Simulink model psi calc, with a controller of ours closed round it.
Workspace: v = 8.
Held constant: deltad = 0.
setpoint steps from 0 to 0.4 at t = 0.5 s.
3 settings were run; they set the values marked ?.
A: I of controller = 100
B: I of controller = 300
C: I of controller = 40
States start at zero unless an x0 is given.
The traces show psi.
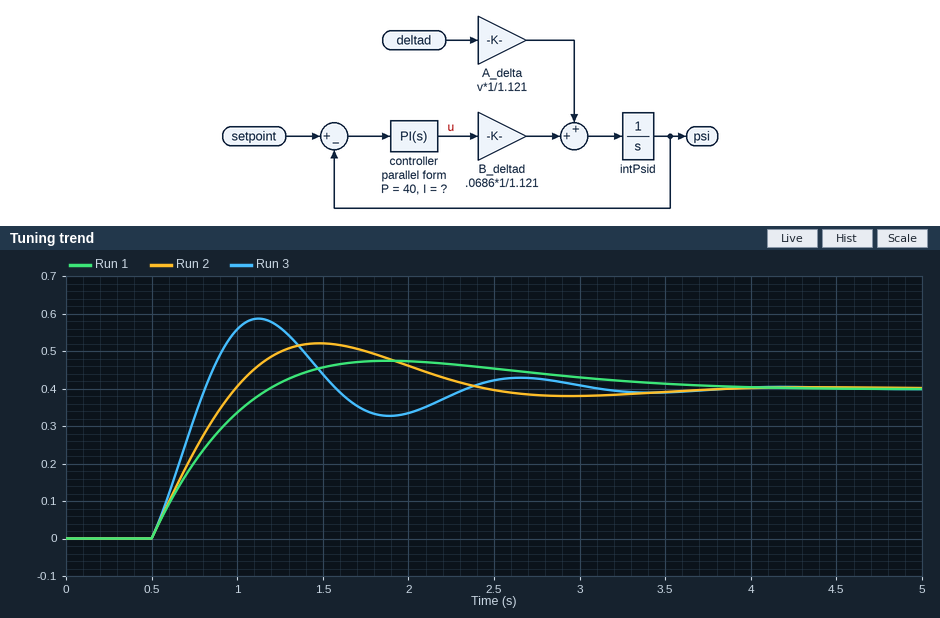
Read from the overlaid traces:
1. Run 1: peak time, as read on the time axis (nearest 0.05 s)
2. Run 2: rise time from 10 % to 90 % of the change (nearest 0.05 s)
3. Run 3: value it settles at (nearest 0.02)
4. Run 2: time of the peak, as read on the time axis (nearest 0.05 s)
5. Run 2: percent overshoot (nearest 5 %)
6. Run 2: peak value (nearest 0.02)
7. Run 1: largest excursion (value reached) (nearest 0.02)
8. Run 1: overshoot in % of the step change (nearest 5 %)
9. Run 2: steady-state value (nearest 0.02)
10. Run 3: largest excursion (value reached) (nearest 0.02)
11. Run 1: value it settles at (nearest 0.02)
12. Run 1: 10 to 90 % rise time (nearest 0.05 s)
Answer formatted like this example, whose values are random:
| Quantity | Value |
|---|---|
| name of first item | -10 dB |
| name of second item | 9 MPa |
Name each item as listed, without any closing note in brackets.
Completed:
| Quantity | Value |
|---|---|
| Run 1: peak time, as read on the time axis | 1.90 s |
| Run 2: rise time from 10 % to 90 % of the change | 0.40 s |
| Run 3: value it settles at | 0.40 |
| Run 2: time of the peak, as read on the time axis | 1.50 s |
| Run 2: percent overshoot | 30 % |
| Run 2: peak value | 0.52 |
| Run 1: largest excursion (value reached) | 0.48 |
| Run 1: overshoot in % of the step change | 20 % |
| Run 2: steady-state value | 0.40 |
| Run 3: largest excursion (value reached) | 0.58 |
| Run 1: value it settles at | 0.40 |
| Run 1: 10 to 90 % rise time | 0.50 s |
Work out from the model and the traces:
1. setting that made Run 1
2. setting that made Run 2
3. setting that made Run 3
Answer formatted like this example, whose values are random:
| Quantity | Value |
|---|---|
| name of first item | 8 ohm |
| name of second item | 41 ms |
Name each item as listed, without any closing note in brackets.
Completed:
| Quantity | Value |
|---|---|
| setting that made Run 1 | C |
| setting that made Run 2 | A |
| setting that made Run 3 | B |
